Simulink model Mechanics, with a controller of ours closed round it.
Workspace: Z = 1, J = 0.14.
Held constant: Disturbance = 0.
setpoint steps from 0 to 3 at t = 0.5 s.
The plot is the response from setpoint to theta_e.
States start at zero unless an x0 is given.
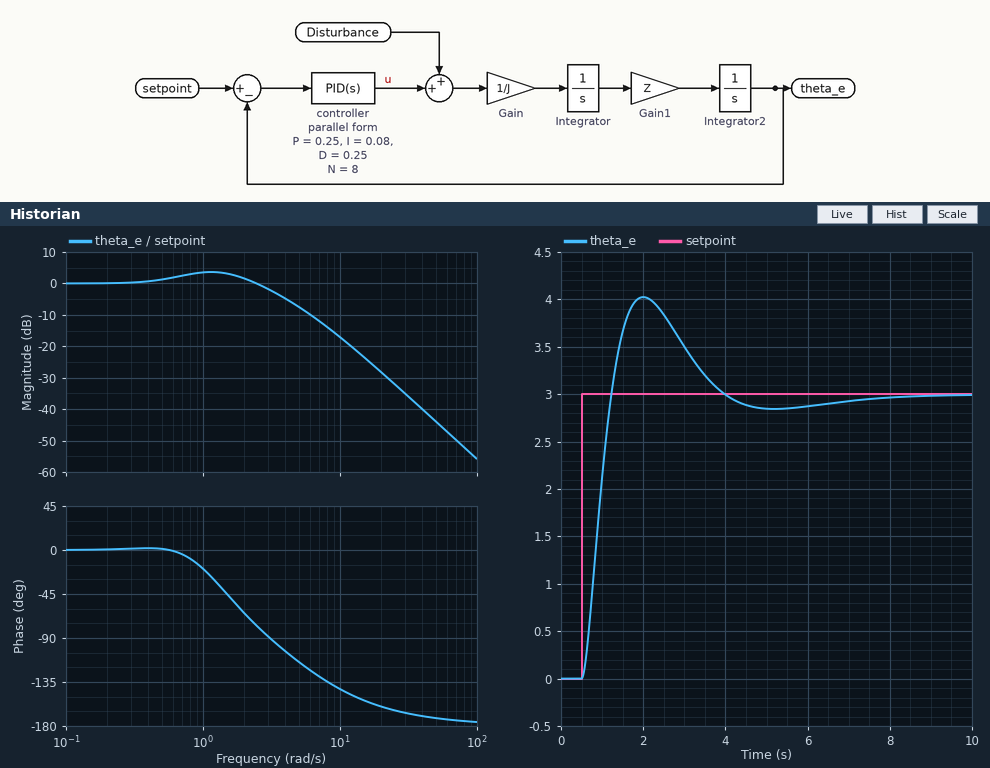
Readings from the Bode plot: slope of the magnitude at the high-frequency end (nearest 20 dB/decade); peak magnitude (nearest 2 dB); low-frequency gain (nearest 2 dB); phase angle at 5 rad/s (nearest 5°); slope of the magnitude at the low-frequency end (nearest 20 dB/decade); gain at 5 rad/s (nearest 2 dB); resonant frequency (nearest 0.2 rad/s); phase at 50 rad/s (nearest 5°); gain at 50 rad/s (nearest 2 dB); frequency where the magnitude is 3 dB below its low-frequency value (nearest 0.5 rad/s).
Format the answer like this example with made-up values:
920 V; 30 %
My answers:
-40 dB/decade; 4 dB; 0 dB; -115°; 0 dB/decade; -8 dB; 1.2 rad/s; -170°; -44 dB; 3.5 rad/s
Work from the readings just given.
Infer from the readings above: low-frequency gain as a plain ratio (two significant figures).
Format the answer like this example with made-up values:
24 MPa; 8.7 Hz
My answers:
1.0
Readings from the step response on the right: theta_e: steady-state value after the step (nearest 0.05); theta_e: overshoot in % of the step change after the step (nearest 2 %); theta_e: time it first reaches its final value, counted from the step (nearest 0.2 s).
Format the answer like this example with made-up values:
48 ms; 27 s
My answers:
3.00; 34 %; 0.8 s
